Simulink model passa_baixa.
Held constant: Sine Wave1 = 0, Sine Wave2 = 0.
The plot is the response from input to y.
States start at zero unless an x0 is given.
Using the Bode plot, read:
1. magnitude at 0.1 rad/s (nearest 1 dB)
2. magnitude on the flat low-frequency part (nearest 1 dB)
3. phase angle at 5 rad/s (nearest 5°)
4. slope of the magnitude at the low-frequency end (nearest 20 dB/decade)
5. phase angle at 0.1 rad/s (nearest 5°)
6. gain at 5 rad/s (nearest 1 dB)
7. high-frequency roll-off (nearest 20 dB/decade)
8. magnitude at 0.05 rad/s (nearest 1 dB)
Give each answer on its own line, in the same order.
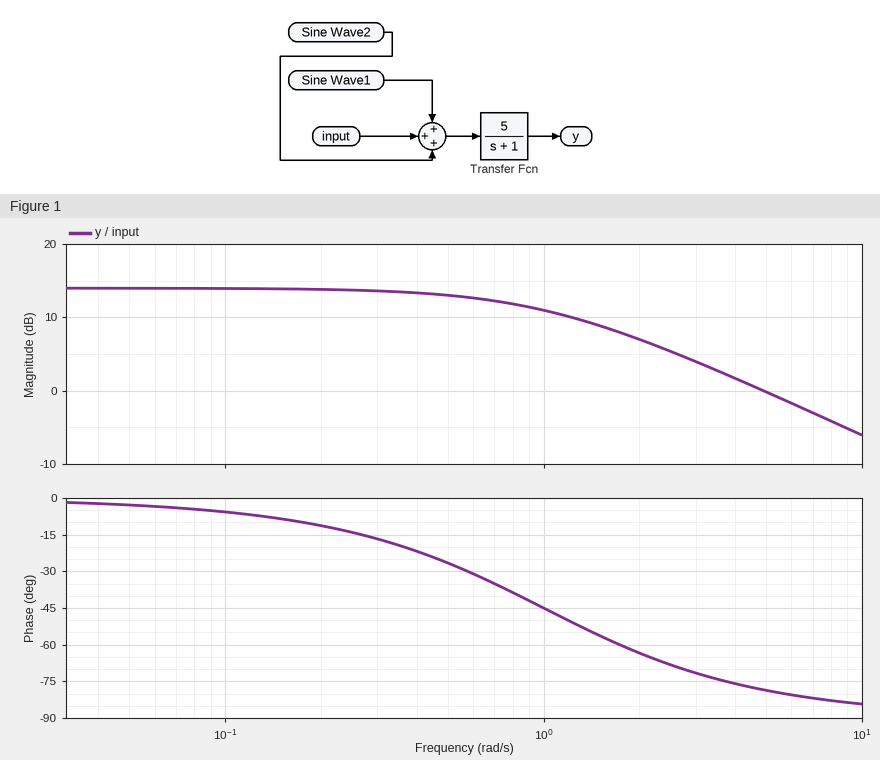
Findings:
14 dB
14 dB
-80°
0 dB/decade
-5°
0 dB
-20 dB/decade
14 dB
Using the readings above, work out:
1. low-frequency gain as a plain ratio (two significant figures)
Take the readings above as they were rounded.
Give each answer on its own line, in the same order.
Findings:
5.0
